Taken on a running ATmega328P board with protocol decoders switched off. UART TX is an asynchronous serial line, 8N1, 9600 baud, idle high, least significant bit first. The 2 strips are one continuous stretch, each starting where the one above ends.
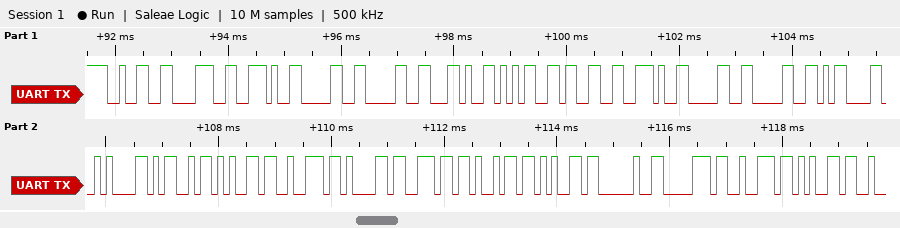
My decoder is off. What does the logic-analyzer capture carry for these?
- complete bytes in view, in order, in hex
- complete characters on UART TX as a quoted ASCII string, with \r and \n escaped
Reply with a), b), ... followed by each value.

a) 0x32 0x38 0x2E 0x30 0x30 0x2C 0x35 0x33 0x2E 0x30 0x30 0x0D 0x0A 0x4D 0x65 0x72 0x61 0x6E 0x69 0x65 0x20 0x70 0x72 0x65
b) "28.00,53.00\r\nMeranie pre"
